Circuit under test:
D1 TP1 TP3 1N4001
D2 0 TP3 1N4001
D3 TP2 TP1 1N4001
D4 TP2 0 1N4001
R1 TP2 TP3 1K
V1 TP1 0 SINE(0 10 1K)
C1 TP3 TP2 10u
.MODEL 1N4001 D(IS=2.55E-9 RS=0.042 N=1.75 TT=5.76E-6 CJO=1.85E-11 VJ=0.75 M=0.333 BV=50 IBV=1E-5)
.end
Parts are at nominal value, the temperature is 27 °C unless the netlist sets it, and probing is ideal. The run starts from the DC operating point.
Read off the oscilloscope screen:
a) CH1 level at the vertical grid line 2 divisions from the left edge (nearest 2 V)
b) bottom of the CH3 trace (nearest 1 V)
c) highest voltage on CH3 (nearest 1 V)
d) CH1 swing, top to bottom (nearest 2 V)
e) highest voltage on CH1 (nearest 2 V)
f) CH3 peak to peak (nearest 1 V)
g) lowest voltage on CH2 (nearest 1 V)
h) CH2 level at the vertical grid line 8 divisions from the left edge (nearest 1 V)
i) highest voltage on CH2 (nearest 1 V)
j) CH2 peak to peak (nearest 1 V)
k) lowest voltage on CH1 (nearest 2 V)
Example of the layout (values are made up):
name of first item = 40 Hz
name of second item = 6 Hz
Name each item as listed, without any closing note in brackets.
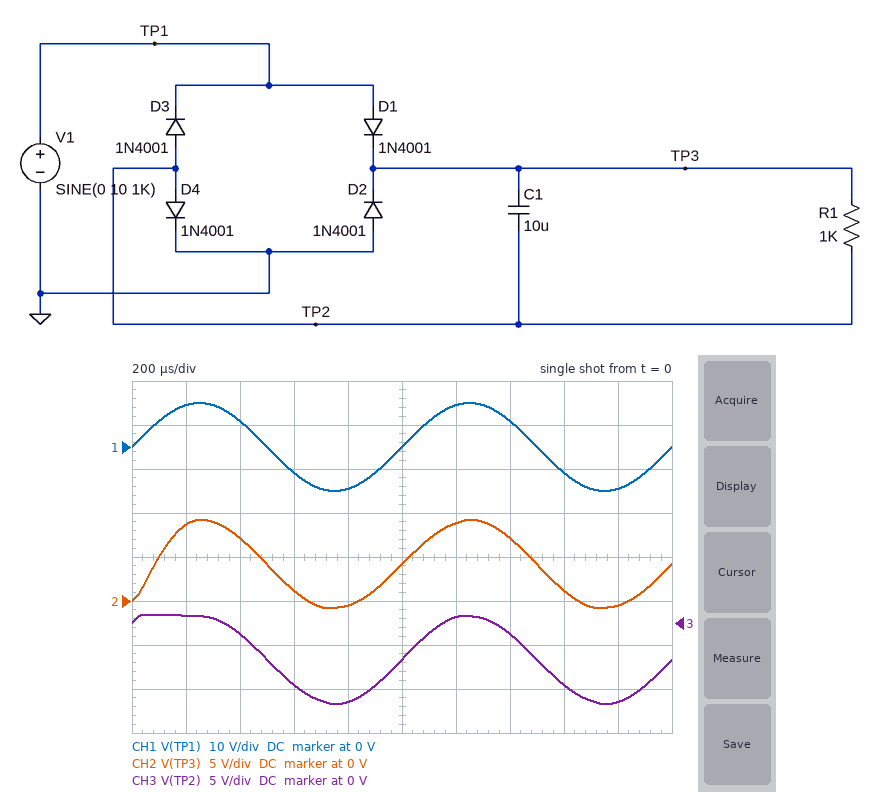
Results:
CH1 level at the vertical grid line 2 divisions from the left edge = 6 V
bottom of the CH3 trace = -9 V
highest voltage on CH3 = 1 V
CH1 swing, top to bottom = 20 V
highest voltage on CH1 = 10 V
CH3 peak to peak = 10 V
lowest voltage on CH2 = -1 V
CH2 level at the vertical grid line 8 divisions from the left edge = 1 V
highest voltage on CH2 = 9 V
CH2 peak to peak = 10 V
lowest voltage on CH1 = -10 V
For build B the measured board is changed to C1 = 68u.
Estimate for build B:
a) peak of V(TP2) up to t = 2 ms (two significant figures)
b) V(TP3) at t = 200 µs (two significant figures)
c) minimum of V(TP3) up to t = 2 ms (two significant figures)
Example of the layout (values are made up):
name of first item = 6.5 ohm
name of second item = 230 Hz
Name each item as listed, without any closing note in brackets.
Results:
peak of V(TP2) up to t = 2 ms = 1.1 V
V(TP3) at t = 200 µs = 8.5 V
minimum of V(TP3) up to t = 2 ms = -830 mV
